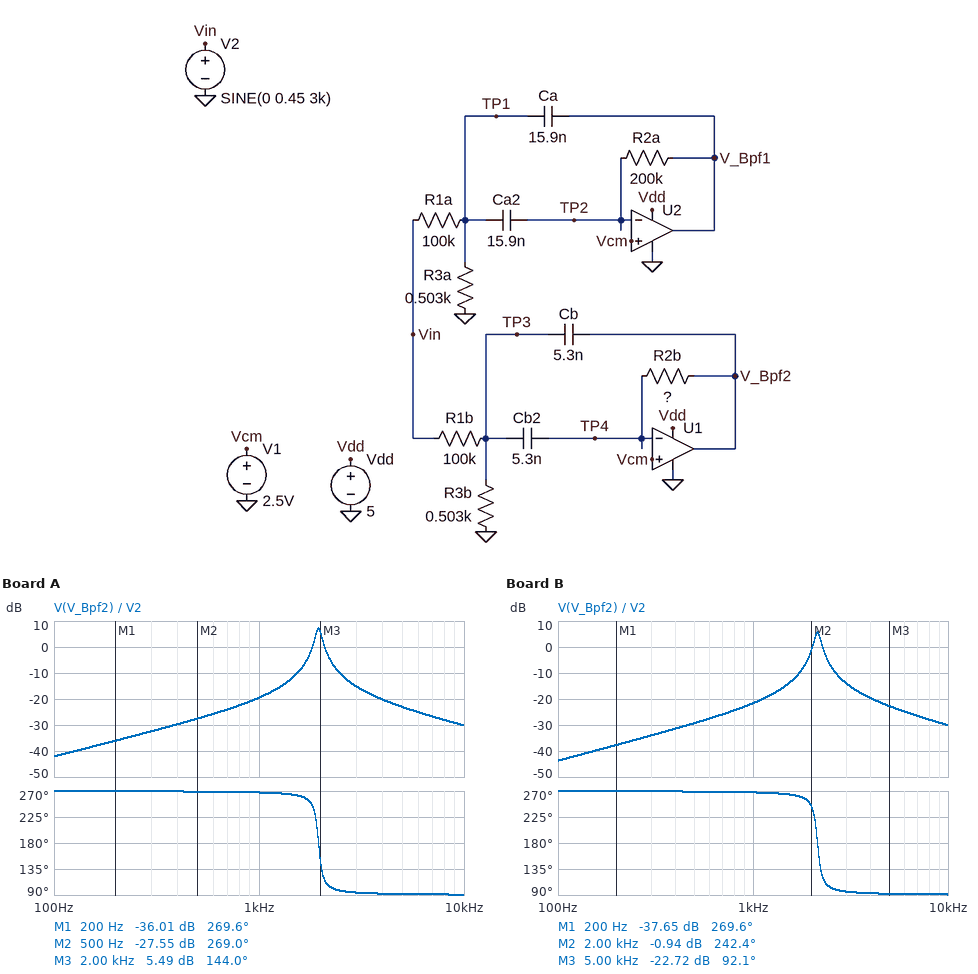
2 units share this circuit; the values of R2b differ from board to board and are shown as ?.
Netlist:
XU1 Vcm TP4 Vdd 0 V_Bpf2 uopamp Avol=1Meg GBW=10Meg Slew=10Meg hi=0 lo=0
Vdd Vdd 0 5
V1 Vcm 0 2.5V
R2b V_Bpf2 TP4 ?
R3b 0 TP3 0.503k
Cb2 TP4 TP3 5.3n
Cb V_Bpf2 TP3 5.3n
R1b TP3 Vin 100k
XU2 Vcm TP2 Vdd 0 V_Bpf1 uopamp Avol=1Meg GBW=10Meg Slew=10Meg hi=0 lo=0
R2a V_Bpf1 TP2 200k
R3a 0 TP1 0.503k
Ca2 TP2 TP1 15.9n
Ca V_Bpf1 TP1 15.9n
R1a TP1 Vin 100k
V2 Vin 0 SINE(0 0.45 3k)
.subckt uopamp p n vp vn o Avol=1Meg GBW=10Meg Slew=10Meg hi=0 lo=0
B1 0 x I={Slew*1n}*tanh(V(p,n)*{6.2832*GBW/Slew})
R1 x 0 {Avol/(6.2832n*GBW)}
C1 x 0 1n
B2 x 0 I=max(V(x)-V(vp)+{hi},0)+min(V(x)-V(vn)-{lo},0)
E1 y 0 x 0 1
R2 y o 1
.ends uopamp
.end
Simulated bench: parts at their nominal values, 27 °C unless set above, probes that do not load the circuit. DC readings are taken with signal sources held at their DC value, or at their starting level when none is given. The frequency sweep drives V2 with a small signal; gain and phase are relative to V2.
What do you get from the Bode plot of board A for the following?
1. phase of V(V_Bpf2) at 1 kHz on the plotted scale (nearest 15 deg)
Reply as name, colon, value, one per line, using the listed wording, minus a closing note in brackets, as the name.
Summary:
phase of V(V_Bpf2) at 1 kHz on the plotted scale: 270 deg
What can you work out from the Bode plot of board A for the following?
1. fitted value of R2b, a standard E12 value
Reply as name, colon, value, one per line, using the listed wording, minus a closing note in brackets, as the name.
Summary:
fitted value of R2b, a standard E12 value: 470 kΩ
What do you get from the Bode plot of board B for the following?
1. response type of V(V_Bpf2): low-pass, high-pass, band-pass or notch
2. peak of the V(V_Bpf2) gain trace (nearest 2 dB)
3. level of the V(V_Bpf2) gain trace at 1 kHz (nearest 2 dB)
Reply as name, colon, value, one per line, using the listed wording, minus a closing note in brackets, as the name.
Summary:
response type of V(V_Bpf2): low-pass, high-pass, band-pass or notch: band-pass
peak of the V(V_Bpf2) gain trace: 6 dB
level of the V(V_Bpf2) gain trace at 1 kHz: -22 dB
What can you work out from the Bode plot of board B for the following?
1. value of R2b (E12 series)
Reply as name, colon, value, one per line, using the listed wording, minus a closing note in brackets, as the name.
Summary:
value of R2b: 390 kΩ
